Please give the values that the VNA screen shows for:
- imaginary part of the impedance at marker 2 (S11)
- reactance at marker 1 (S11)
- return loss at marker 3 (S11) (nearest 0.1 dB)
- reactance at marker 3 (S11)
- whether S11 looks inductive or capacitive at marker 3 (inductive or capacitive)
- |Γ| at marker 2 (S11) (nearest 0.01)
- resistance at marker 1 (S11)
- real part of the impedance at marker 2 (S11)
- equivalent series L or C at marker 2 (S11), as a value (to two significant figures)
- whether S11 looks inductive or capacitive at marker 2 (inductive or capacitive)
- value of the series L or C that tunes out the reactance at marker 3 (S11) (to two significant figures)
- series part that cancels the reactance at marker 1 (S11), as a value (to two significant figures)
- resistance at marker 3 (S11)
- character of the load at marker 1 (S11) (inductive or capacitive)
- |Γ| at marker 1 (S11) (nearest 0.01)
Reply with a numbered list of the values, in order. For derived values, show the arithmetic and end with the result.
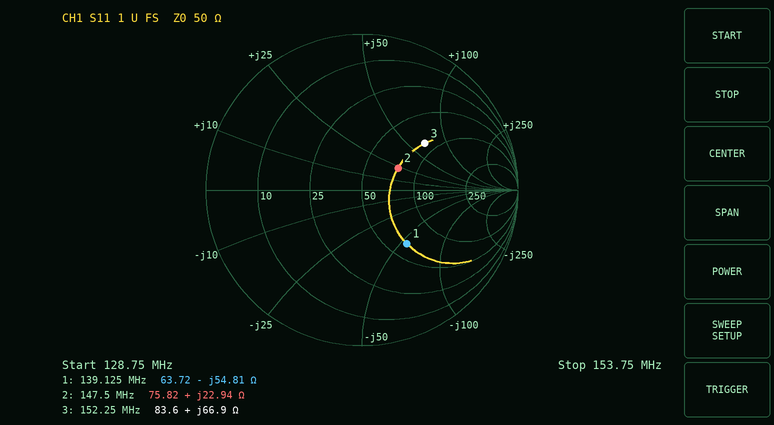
1. +22.94 Ω
2. -54.81 Ω
3. 6.0 dB
4. +66.9 Ω
5. inductive
6. 0.27
7. 63.72 Ω
8. 75.82 Ω
9. L = 22.94 Ω/(2π × 147.5 MHz) ≈ 25 nH
10. inductive
11. C = 1/(2π × 152.25 MHz × 66.9 Ω) ≈ 16 pF
12. L = 54.81 Ω/(2π × 139.125 MHz) ≈ 63 nH
13. 83.6 Ω
14. capacitive
15. 0.45
